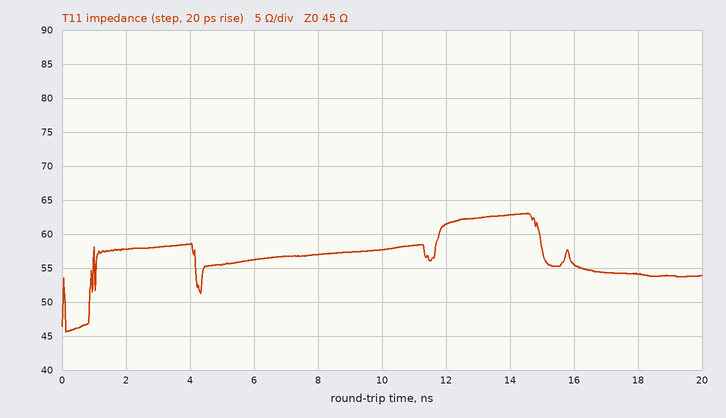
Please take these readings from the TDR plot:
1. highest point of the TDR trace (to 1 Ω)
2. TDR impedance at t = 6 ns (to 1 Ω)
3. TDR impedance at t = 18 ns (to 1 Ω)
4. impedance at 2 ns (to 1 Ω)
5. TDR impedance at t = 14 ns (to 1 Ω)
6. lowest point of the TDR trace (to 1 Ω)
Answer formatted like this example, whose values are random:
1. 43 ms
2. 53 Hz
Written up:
1. 63 Ω
2. 56 Ω
3. 54 Ω
4. 58 Ω
5. 63 Ω
6. 46 Ω
